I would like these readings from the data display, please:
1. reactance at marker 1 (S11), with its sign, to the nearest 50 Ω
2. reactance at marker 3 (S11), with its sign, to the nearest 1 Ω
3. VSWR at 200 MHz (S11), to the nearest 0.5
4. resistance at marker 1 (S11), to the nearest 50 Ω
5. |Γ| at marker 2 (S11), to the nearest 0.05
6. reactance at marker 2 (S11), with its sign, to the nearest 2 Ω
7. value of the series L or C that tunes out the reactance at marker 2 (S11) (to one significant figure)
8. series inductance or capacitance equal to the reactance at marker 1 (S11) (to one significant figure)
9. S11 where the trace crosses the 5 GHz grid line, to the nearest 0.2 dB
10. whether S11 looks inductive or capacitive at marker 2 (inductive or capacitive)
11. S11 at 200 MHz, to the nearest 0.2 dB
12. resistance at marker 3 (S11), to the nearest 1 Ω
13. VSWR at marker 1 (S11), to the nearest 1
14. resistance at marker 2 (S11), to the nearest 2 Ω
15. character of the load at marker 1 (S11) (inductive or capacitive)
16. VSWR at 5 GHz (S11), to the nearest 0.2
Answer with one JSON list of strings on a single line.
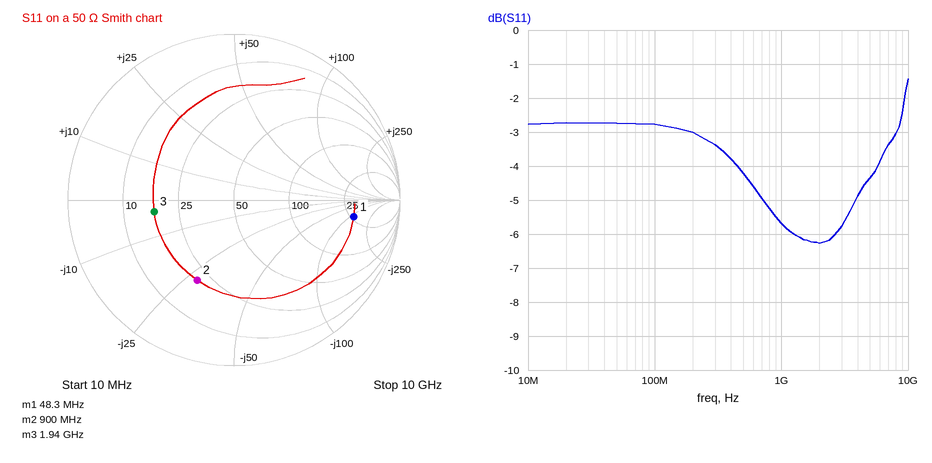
["-100 Ω", "-3 Ω", "6.0", "250 Ω", "0.55", "-28 Ω", "5 nH", "30 pF", "-4.4 dB", "capacitive", "-3.0 dB", "17 Ω", "6", "20 Ω", "capacitive", "4.0"]
